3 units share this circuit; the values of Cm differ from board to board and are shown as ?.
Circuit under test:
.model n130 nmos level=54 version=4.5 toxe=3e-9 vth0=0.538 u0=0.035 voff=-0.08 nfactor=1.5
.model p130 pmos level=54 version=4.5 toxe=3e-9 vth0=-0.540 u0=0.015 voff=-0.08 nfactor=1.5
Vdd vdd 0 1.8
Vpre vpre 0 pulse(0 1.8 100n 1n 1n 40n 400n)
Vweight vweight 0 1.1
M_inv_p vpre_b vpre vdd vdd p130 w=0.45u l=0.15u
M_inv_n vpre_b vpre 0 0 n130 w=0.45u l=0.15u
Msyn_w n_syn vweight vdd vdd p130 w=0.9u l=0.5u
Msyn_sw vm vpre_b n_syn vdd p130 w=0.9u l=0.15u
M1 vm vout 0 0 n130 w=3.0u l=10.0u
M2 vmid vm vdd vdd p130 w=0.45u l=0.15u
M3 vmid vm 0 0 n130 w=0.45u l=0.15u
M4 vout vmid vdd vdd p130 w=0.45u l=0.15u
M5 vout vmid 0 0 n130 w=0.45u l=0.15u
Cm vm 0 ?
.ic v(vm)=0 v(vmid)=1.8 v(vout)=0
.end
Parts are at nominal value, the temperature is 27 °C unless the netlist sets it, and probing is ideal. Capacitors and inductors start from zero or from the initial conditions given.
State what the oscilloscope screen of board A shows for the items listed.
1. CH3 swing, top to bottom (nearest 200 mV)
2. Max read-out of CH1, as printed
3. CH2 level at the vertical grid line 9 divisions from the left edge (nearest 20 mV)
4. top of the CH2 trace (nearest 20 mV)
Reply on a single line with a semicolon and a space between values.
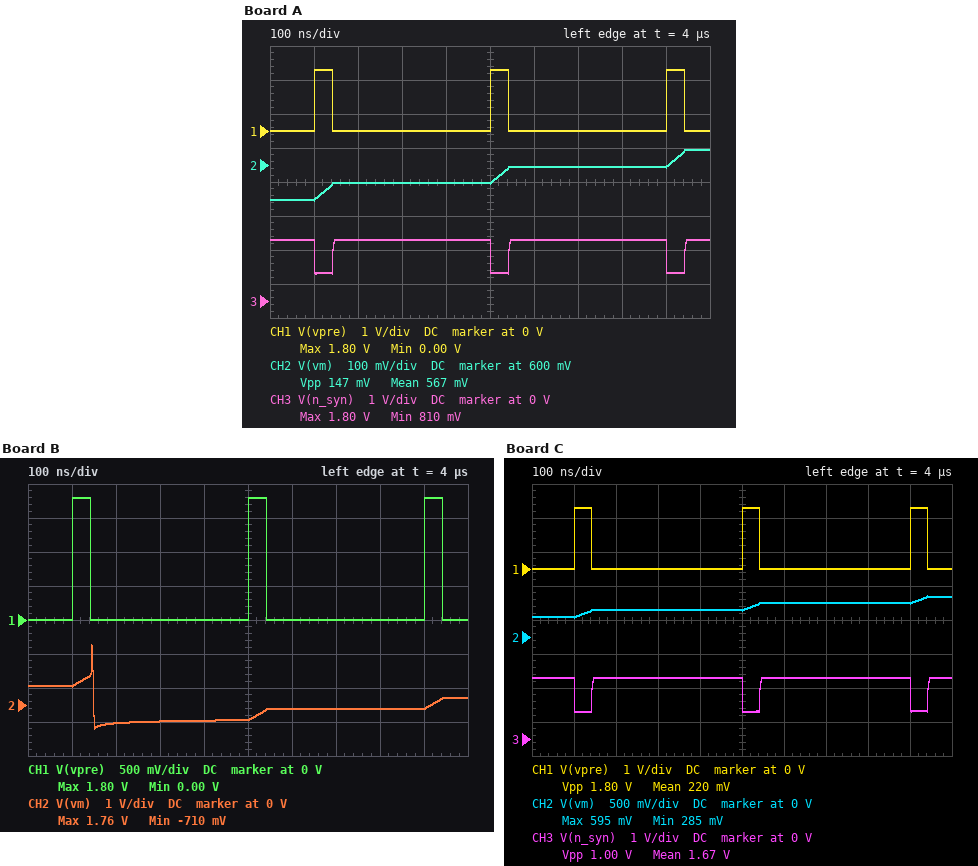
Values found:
1.0 V; 1.80 V; 600 mV; 640 mV
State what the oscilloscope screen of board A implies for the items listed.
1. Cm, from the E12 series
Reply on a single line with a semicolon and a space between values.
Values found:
390 fF
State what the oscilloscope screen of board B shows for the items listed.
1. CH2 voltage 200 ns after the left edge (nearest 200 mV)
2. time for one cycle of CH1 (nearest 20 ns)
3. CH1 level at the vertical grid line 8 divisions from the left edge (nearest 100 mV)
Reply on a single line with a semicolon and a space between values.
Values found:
-600 mV; 400 ns; 0 V
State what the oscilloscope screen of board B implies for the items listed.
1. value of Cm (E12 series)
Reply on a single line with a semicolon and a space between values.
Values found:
47 fF
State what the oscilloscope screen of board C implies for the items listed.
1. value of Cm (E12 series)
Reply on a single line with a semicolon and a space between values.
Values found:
180 fF
